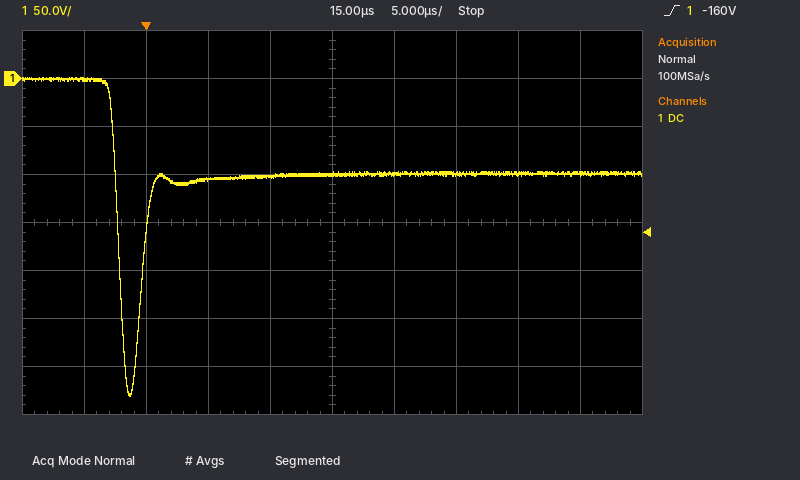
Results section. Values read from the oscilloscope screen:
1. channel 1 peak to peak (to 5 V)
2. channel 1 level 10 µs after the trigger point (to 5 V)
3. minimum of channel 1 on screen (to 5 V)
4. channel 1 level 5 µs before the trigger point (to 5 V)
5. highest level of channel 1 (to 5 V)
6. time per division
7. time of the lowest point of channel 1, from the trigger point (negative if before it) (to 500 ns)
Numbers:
330 V
-100 V
-330 V
0 V
0 V
5 µs
-1.5 µs
